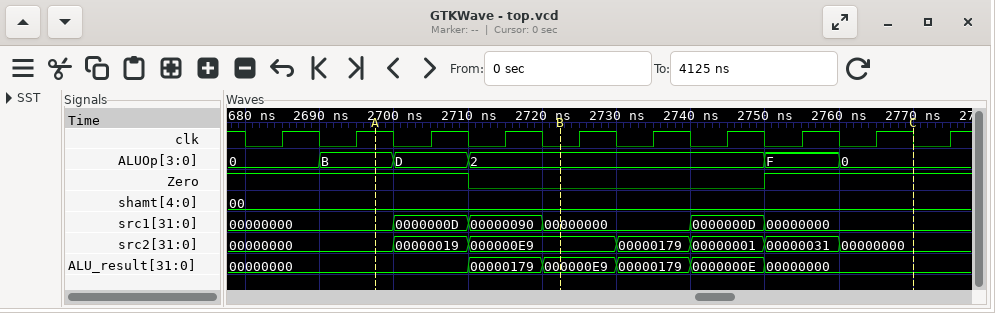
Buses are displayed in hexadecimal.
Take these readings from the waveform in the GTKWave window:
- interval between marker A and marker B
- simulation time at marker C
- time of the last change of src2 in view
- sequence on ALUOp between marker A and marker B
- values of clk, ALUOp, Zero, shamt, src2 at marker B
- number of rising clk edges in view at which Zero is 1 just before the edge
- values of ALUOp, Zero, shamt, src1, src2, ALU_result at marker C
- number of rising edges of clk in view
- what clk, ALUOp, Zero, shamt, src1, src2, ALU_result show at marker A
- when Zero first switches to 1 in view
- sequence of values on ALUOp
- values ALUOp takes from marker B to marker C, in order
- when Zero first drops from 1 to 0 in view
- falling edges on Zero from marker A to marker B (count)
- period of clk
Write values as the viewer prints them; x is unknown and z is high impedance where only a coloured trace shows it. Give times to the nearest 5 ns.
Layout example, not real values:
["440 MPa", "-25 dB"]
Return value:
["25 ns", "2770 ns", "2760 ns", "B, D, 2", "clk=0, ALUOp=2, Zero=0, shamt=00, src2=000000E9", "6", "ALUOp=0, Zero=1, shamt=00, src1=00000000, src2=00000000, ALU_result=00000000", "10", "clk=1, ALUOp=B, Zero=1, shamt=00, src1=00000000, src2=00000000, ALU_result=00000000", "2750 ns", "0, B, D, 2, F, 0", "2, F, 0", "2710 ns", "1", "10 ns"]
